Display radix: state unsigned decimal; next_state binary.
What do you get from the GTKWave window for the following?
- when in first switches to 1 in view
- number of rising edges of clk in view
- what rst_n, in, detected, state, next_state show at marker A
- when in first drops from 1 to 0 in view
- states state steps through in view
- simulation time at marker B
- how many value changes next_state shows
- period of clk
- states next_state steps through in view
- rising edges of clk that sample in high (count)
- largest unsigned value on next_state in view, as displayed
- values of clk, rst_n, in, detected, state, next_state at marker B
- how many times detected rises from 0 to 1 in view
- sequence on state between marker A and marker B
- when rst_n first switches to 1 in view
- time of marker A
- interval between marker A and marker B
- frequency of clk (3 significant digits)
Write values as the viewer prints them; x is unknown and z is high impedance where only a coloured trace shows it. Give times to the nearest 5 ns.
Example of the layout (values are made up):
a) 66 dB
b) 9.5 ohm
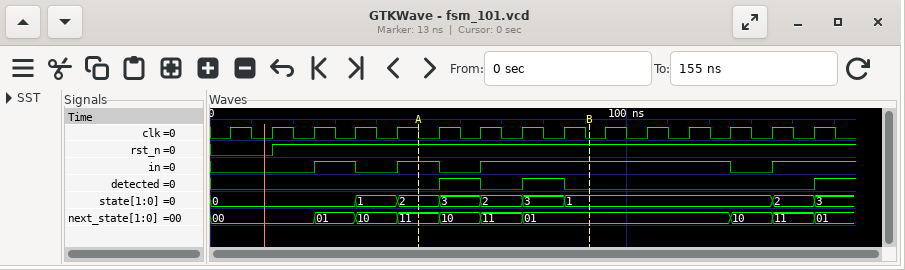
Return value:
a) 25 ns
b) 15
c) rst_n=1, in=1, detected=0, state=2, next_state=11
d) 35 ns
e) 0, 1, 2, 3, 2, 3, 1, 2, 3
f) 90 ns
g) 9
h) 10 ns
i) 00, 01, 10, 11, 10, 11, 01, 10, 11, 01
j) 9
k) 11
l) clk=0, rst_n=1, in=1, detected=0, state=1, next_state=01
m) 3
n) 2, 3, 2, 3, 1
o) 15 ns
p) 50 ns
q) 40 ns
r) 100 MHz
